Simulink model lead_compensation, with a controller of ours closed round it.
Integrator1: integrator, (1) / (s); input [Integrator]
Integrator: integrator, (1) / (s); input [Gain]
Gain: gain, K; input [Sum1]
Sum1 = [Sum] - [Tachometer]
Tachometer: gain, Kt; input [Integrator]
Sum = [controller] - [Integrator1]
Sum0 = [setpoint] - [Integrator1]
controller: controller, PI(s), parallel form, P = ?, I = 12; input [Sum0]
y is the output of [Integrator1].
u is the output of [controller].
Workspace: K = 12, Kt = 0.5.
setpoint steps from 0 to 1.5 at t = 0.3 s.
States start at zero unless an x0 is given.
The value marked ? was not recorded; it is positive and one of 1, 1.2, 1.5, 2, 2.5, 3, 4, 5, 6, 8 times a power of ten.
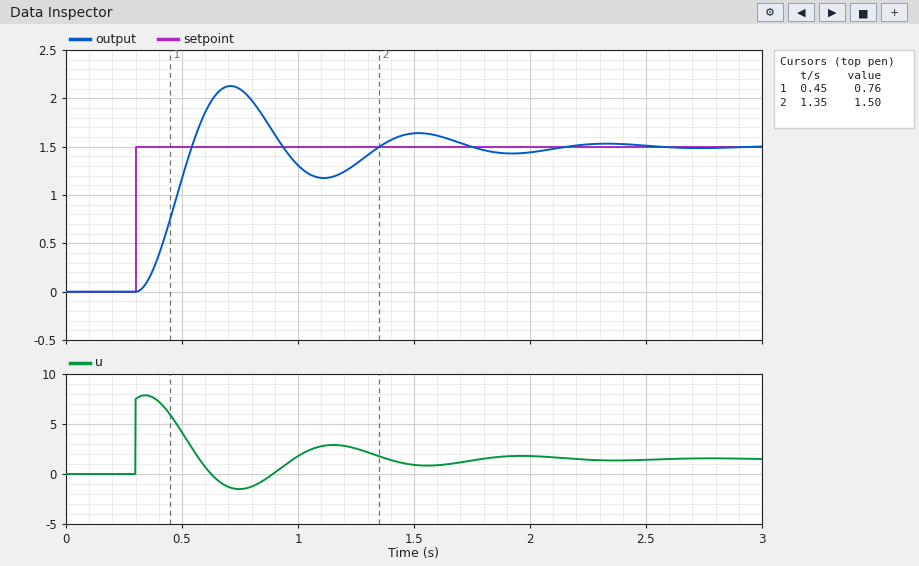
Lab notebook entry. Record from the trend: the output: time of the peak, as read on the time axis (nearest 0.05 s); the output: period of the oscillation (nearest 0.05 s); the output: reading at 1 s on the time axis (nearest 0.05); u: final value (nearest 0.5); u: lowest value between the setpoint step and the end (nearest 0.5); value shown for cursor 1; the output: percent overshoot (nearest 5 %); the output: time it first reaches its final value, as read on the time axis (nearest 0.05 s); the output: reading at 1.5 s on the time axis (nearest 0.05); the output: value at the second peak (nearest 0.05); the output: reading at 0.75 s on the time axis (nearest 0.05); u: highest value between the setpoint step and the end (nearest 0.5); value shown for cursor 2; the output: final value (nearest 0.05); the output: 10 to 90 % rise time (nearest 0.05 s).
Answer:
0.70 s
0.80 s
1.30
1.5
-1.5
0.76
40 %
0.55 s
1.65
1.65
2.10
8.0
1.50
1.50
0.15 s
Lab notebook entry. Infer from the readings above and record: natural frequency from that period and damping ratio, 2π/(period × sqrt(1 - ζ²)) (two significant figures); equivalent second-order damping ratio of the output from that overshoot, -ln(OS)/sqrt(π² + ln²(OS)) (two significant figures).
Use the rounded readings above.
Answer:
8.2 rad/s
0.28
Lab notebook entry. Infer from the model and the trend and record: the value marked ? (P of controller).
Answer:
5
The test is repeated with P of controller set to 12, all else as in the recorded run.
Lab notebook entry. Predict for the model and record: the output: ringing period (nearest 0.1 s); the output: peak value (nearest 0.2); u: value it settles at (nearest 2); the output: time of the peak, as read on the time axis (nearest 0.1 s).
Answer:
0.5 s
2.2
2
0.6 s
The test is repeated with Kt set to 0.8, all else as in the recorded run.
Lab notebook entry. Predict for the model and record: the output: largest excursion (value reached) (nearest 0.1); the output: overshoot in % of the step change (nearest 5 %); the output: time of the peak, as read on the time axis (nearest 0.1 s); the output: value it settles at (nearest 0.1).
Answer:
1.9
25 %
0.8 s
1.5
